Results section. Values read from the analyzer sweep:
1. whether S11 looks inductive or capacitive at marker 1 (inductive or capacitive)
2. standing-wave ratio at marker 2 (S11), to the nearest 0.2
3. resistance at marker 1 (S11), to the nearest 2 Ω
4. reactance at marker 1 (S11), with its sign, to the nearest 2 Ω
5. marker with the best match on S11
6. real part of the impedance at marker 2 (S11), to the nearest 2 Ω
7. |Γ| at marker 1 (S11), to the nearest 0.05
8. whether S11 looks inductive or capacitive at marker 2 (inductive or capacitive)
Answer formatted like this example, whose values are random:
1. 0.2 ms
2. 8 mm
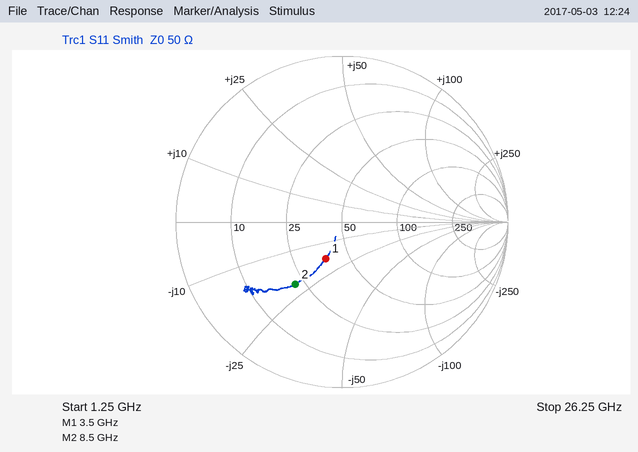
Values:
1. capacitive
2. 2.8
3. 38 Ω
4. -18 Ω
5. marker 1
6. 22 Ω
7. 0.25
8. capacitive
